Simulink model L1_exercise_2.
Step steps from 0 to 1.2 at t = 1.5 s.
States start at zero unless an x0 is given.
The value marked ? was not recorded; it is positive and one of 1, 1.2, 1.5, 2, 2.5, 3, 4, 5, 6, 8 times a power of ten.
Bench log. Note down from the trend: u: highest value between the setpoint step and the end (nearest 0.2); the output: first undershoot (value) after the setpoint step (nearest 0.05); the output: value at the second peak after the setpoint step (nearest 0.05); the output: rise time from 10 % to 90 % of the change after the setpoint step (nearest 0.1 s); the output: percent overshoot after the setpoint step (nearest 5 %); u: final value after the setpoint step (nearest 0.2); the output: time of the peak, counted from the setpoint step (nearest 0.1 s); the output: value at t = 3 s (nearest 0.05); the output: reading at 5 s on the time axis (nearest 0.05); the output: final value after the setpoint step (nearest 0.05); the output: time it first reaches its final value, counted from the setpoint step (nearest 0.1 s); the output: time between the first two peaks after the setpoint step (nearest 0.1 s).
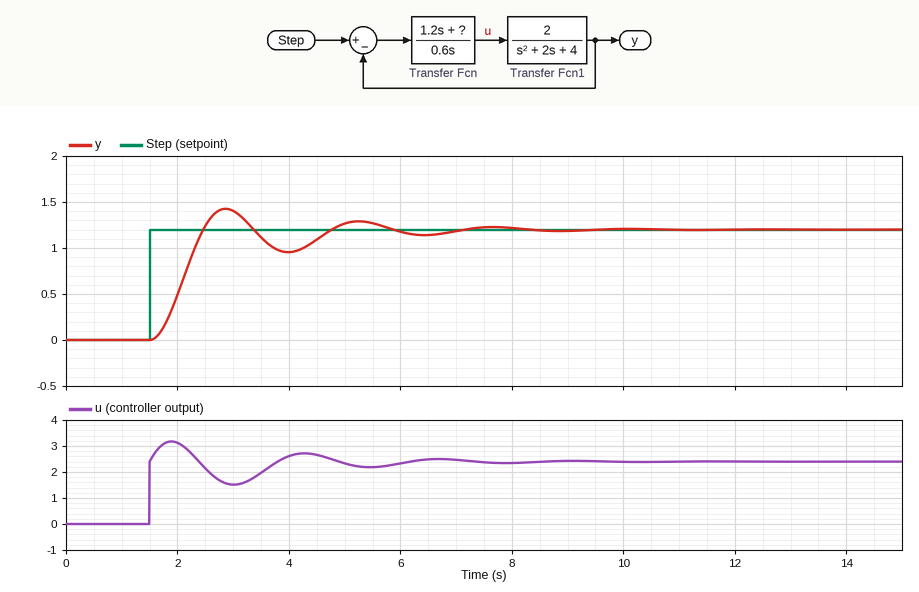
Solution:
3.2
0.95
1.30
0.6 s
20 %
2.4
1.4 s
1.40
1.25
1.20
1.0 s
2.4 s
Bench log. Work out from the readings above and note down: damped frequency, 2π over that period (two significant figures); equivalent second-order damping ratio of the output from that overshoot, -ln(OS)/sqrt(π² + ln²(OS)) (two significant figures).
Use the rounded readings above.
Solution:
2.6 rad/s
0.46
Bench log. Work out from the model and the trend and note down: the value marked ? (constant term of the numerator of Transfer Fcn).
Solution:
2
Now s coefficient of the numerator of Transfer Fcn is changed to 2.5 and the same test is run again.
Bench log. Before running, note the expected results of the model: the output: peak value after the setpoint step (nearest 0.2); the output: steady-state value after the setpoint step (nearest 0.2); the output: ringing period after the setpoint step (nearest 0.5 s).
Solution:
1.4
1.2
2.0 s
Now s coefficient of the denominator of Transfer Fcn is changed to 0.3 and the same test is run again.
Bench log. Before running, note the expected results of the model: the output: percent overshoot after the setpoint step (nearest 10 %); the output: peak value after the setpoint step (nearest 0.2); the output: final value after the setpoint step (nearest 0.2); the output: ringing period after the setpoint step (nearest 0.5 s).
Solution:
40 %
1.8
1.2
2.0 s
